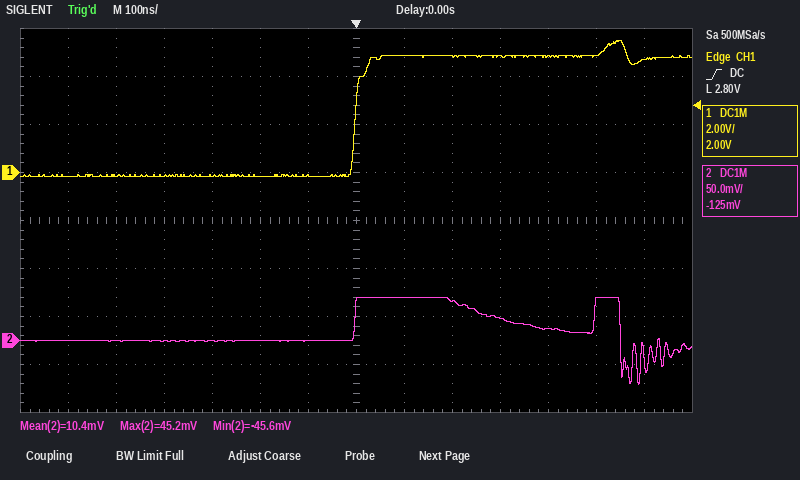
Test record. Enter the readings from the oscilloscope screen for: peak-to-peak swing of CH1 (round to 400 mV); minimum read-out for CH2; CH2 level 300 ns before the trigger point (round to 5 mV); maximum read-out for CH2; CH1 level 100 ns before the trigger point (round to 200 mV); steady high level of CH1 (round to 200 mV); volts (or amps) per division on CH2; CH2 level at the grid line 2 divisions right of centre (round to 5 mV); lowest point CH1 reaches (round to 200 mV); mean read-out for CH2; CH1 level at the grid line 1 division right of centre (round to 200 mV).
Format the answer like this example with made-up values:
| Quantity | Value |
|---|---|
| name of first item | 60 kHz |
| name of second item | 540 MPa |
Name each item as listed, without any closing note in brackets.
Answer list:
| Quantity | Value |
|---|---|
| peak-to-peak swing of CH1 | 5.6 V |
| minimum read-out for CH2 | -45.6 mV |
| CH2 level 300 ns before the trigger point | 0 mV |
| maximum read-out for CH2 | 45.2 mV |
| CH1 level 100 ns before the trigger point | -200 mV |
| steady high level of CH1 | 4.8 V |
| volts (or amps) per division on CH2 | 50 mV |
| CH2 level at the grid line 2 divisions right of centre | 40 mV |
| lowest point CH1 reaches | -200 mV |
| mean read-out for CH2 | 10.4 mV |
| CH1 level at the grid line 1 division right of centre | 4.8 V |
